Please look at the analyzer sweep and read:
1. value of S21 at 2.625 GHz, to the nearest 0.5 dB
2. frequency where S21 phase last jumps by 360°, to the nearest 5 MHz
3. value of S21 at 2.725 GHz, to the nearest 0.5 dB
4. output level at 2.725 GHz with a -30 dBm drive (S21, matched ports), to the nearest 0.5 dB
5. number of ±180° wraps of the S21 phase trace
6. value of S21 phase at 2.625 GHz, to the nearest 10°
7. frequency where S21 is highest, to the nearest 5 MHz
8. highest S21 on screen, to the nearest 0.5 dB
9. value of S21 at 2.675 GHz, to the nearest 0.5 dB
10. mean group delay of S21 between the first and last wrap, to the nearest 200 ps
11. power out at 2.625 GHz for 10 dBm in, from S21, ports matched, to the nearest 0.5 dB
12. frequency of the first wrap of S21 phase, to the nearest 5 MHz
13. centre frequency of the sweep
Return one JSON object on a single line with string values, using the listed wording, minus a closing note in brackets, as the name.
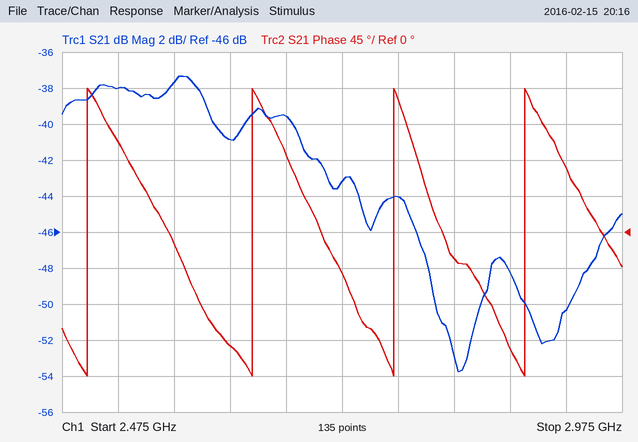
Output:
{"value of S21 at 2.625 GHz, to the nearest 0.5 dB": "-41.0 dB", "frequency where S21 phase last jumps by 360°, to the nearest 5 MHz": "2.890 GHz", "value of S21 at 2.725 GHz, to the nearest 0.5 dB": "-43.0 dB", "output level at 2.725 GHz with a -30 dBm drive (S21, matched ports), to the nearest 0.5 dB": "-73.0 dBm", "number of ±180° wraps of the S21 phase trace": "4", "value of S21 phase at 2.625 GHz, to the nearest 10°": "-140°", "frequency where S21 is highest, to the nearest 5 MHz": "2.580 GHz", "highest S21 on screen, to the nearest 0.5 dB": "-37.5 dB", "value of S21 at 2.675 GHz, to the nearest 0.5 dB": "-39.5 dB", "mean group delay of S21 between the first and last wrap, to the nearest 200 ps": "7.6 ns", "power out at 2.625 GHz for 10 dBm in, from S21, ports matched, to the nearest 0.5 dB": "-31.0 dBm", "frequency of the first wrap of S21 phase, to the nearest 5 MHz": "2.500 GHz", "centre frequency of the sweep": "2.725 GHz"}
